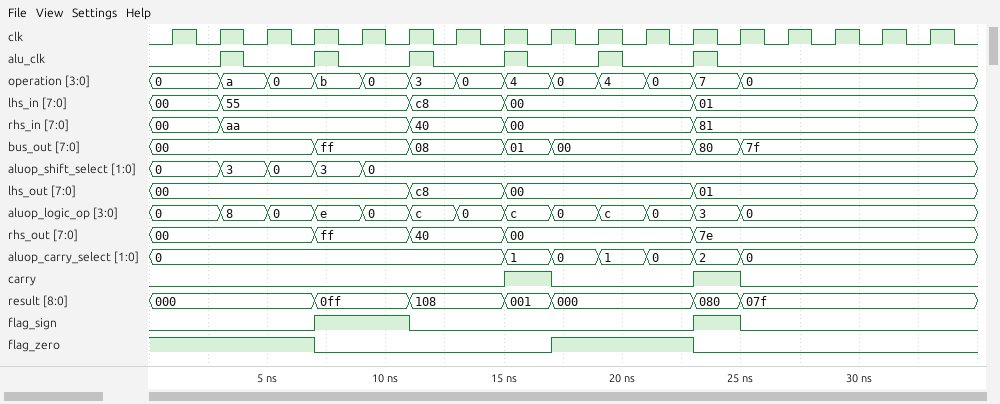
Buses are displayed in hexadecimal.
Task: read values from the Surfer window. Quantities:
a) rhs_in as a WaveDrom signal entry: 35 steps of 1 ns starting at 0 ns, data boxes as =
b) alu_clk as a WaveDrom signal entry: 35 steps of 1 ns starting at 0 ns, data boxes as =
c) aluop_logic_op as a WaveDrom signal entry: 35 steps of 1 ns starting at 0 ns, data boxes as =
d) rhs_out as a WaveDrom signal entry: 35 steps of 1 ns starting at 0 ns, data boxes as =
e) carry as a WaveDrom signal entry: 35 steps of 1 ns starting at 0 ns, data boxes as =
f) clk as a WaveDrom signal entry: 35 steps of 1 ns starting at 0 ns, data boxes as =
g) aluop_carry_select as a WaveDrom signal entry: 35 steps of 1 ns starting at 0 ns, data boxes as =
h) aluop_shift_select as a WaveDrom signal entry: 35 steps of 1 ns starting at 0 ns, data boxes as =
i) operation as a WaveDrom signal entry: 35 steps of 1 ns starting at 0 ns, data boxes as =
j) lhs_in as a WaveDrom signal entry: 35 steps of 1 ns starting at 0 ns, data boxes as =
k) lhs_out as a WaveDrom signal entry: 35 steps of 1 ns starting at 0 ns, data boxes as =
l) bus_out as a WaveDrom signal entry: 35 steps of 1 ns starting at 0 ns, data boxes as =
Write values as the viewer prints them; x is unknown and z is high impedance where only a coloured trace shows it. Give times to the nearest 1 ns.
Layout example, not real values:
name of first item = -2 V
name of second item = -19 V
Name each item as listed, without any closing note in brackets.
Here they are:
rhs_in as a WaveDrom signal entry: 35 steps of 1 ns starting at 0 ns, data boxes as = = {name: 'rhs_in', wave: '=..=.......=...=.......=...........', data: '00 aa 40 00 81'}
alu_clk as a WaveDrom signal entry: 35 steps of 1 ns starting at 0 ns, data boxes as = = {name: 'alu_clk', wave: '0..10..10..10..10..10..10..........'}
aluop_logic_op as a WaveDrom signal entry: 35 steps of 1 ns starting at 0 ns, data boxes as = = {name: 'aluop_logic_op', wave: '=..=.=.=.=.=.=.=.=.=.=.=.=.........', data: '0 8 0 e 0 c 0 c 0 c 0 3 0'}
rhs_out as a WaveDrom signal entry: 35 steps of 1 ns starting at 0 ns, data boxes as = = {name: 'rhs_out', wave: '=......=...=...=.......=...........', data: '00 ff 40 00 7e'}
carry as a WaveDrom signal entry: 35 steps of 1 ns starting at 0 ns, data boxes as = = {name: 'carry', wave: '0..............1.0.....1.0.........'}
clk as a WaveDrom signal entry: 35 steps of 1 ns starting at 0 ns, data boxes as = = {name: 'clk', wave: '01010101010101010101010101010101010'}
aluop_carry_select as a WaveDrom signal entry: 35 steps of 1 ns starting at 0 ns, data boxes as = = {name: 'aluop_carry_select', wave: '=..............=.=.=.=.=.=.........', data: '0 1 0 1 0 2 0'}
aluop_shift_select as a WaveDrom signal entry: 35 steps of 1 ns starting at 0 ns, data boxes as = = {name: 'aluop_shift_select', wave: '=..=.=.=.=.........................', data: '0 3 0 3 0'}
operation as a WaveDrom signal entry: 35 steps of 1 ns starting at 0 ns, data boxes as = = {name: 'operation', wave: '=..=.=.=.=.=.=.=.=.=.=.=.=.........', data: '0 a 0 b 0 3 0 4 0 4 0 7 0'}
lhs_in as a WaveDrom signal entry: 35 steps of 1 ns starting at 0 ns, data boxes as = = {name: 'lhs_in', wave: '=..=.......=...=.......=...........', data: '00 55 c8 00 01'}
lhs_out as a WaveDrom signal entry: 35 steps of 1 ns starting at 0 ns, data boxes as = = {name: 'lhs_out', wave: '=..........=...=.......=...........', data: '00 c8 00 01'}
bus_out as a WaveDrom signal entry: 35 steps of 1 ns starting at 0 ns, data boxes as = = {name: 'bus_out', wave: '=......=...=...=.=.....=.=.........', data: '00 ff 08 01 00 80 7f'}
